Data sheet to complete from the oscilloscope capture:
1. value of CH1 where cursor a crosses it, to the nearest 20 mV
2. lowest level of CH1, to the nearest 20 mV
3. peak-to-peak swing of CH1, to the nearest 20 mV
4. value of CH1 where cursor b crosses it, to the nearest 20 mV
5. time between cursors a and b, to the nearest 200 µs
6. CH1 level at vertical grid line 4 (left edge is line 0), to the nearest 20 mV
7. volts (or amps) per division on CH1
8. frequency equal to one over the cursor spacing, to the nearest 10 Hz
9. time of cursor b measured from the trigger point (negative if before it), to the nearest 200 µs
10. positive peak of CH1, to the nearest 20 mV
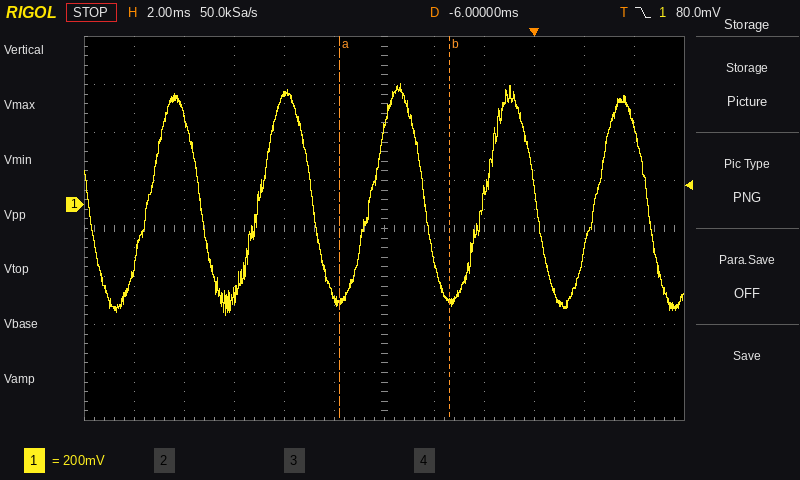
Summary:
-400 mV
-460 mV
960 mV
-400 mV
4.4 ms
460 mV
200 mV
230 Hz
-3.4 ms
500 mV
